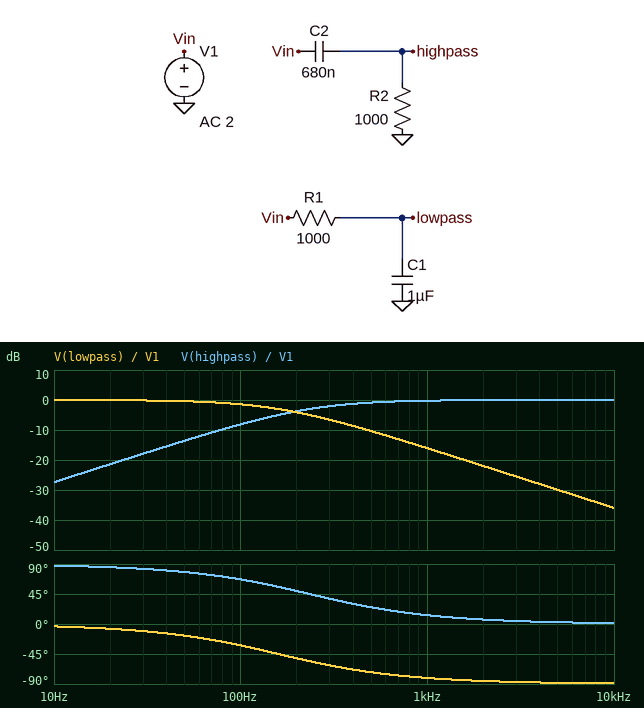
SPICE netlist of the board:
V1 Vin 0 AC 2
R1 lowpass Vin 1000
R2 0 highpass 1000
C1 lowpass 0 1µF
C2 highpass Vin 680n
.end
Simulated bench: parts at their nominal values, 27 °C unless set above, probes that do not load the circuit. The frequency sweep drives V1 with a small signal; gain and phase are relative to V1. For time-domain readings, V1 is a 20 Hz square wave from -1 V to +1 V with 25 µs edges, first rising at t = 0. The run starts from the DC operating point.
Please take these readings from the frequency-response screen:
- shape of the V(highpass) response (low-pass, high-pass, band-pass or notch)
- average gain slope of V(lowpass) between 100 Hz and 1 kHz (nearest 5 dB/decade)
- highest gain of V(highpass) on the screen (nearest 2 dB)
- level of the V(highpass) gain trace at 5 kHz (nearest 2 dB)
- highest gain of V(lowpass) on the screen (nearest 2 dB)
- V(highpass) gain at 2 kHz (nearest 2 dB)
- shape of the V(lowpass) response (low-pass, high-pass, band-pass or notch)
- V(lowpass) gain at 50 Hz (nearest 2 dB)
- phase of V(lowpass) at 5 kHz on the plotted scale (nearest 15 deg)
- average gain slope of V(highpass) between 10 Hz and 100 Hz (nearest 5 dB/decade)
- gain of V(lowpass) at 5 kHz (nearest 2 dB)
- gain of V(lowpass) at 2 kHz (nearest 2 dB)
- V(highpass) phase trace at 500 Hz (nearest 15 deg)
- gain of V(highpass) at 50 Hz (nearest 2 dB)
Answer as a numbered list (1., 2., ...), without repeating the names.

1. high-pass
2. -15 dB/decade
3. 0 dB
4. 0 dB
5. 0 dB
6. 0 dB
7. low-pass
8. 0 dB
9. -90 deg
10. 20 dB/decade
11. -30 dB
12. -22 dB
13. 30 deg
14. -14 dB
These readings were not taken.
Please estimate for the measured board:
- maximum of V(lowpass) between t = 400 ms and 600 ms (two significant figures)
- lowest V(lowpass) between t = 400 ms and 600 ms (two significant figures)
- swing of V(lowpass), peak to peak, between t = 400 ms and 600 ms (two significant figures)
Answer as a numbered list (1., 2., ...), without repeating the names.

1. 1.0 V
2. -1.0 V
3. 2.0 V
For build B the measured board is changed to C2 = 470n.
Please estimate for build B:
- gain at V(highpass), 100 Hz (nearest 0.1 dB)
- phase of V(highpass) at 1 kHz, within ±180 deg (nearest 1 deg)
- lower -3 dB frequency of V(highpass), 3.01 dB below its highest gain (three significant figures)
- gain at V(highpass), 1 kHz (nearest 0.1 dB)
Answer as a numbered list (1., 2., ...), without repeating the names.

1. -11.0 dB
2. 19 deg
3. 339 Hz
4. -0.5 dB
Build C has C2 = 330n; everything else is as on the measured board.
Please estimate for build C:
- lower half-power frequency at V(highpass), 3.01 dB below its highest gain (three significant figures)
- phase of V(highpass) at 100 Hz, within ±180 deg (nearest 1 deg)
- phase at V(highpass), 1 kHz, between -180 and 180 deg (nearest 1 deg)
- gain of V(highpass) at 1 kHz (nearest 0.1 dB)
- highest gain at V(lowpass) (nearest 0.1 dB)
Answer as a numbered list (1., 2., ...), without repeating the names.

1. 482 Hz
2. 78 deg
3. 26 deg
4. -0.9 dB
5. 0 dB
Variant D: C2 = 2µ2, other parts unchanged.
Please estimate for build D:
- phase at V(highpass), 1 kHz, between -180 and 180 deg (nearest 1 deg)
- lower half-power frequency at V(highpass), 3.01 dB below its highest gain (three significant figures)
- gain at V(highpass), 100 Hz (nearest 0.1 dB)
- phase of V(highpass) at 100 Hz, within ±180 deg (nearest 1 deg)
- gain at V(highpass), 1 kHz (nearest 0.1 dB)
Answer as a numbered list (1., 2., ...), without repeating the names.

1. 4 deg
2. 72.3 Hz
3. -1.8 dB
4. 36 deg
5. 0 dB
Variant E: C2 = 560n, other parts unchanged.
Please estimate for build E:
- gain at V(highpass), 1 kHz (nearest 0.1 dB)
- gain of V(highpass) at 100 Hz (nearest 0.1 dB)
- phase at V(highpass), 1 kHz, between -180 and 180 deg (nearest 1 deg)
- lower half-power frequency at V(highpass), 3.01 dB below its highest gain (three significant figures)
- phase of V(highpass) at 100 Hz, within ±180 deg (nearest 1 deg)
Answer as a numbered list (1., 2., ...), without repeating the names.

1. -0.3 dB
2. -9.6 dB
3. 16 deg
4. 284 Hz
5. 71 deg
